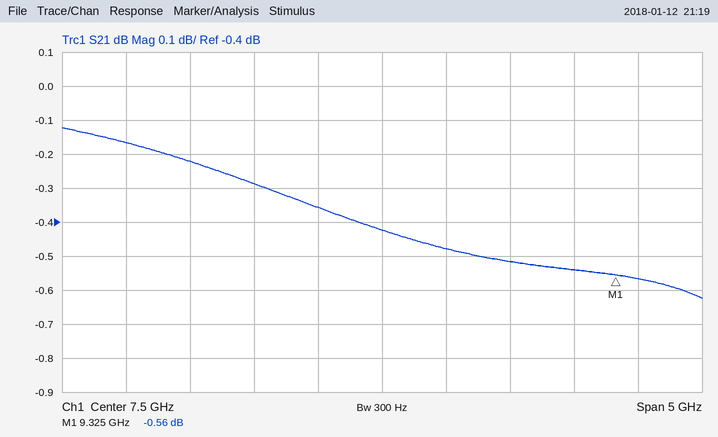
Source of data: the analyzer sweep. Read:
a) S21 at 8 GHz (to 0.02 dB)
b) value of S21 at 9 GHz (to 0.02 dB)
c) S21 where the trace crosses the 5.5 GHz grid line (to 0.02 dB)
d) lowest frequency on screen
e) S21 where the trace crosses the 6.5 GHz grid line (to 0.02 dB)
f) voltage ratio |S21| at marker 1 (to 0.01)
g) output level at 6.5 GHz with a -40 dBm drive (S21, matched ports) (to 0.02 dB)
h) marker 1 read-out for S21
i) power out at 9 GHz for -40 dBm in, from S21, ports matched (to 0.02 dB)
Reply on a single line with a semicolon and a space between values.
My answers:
-0.48 dB; -0.54 dB; -0.16 dB; 5 GHz; -0.28 dB; 0.94; -40.28 dBm; -0.56 dB; -40.54 dBm
